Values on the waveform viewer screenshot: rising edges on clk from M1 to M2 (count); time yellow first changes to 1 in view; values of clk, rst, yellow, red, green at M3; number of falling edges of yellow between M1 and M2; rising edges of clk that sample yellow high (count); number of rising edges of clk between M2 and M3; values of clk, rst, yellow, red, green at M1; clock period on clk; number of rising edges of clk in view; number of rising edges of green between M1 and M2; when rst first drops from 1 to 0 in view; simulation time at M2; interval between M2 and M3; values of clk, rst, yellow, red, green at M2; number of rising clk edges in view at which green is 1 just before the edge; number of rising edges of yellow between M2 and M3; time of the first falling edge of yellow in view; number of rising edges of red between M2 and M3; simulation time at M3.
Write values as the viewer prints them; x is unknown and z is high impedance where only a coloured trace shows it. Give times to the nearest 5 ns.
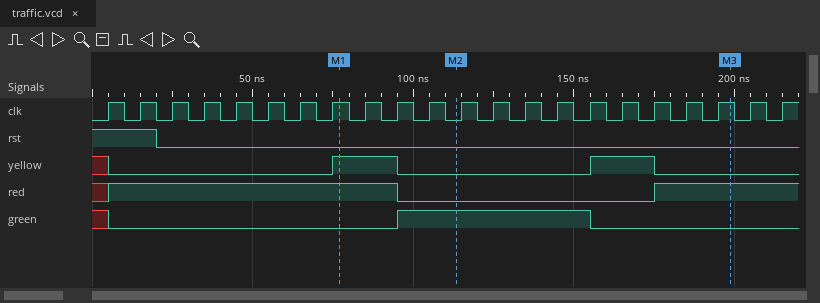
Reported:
3
75 ns
clk=1, rst=0, yellow=0, red=1, green=0
1
4
9
clk=1, rst=0, yellow=1, red=1, green=0
10 ns
22
1
20 ns
115 ns
85 ns
clk=0, rst=0, yellow=0, red=0, green=1
6
1
95 ns
1
200 ns
